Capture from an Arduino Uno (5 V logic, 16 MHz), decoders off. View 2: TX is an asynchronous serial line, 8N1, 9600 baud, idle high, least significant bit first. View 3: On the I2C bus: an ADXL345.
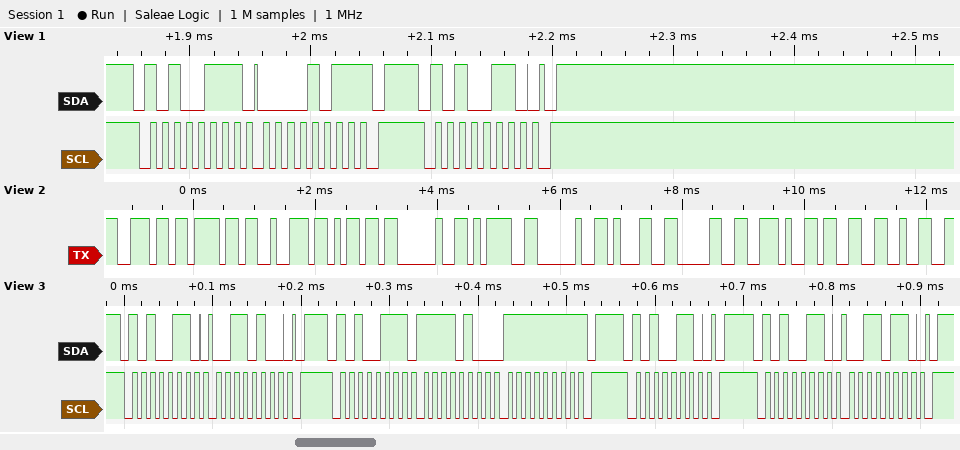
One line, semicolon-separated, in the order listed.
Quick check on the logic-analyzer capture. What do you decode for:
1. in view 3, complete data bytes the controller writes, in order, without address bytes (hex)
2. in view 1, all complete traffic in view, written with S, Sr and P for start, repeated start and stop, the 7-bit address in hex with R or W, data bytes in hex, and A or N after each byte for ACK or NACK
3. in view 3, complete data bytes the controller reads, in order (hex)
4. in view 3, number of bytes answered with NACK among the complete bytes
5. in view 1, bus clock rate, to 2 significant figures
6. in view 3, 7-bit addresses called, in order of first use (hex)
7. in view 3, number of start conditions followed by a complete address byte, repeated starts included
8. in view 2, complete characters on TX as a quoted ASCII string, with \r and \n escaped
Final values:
34 36; S 53R A 0B N P S 53W A P; F4 FF; 1; 100 kHz; 0x53; 4; "norm = 10.32"
